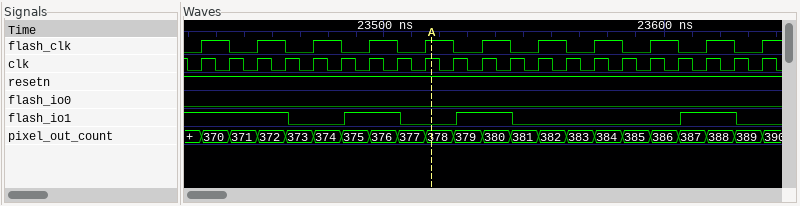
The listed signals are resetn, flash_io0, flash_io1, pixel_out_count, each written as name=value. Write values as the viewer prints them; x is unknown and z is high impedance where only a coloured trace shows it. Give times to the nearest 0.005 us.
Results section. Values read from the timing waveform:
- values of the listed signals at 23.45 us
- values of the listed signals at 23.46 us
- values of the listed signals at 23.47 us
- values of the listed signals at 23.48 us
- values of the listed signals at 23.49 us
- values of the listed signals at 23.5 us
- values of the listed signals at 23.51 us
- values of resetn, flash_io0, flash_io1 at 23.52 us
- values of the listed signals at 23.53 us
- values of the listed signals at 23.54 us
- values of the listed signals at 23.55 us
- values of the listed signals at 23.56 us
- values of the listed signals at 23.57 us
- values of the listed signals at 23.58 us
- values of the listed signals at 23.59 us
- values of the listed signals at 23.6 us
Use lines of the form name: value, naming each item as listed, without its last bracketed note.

values of the listed signals at 23.45 us: resetn=1, flash_io0=0, flash_io1=1, pixel_out_count=371
values of the listed signals at 23.46 us: resetn=1, flash_io0=0, flash_io1=1, pixel_out_count=372
values of the listed signals at 23.47 us: resetn=1, flash_io0=0, flash_io1=0, pixel_out_count=373
values of the listed signals at 23.48 us: resetn=1, flash_io0=0, flash_io1=0, pixel_out_count=374
values of the listed signals at 23.49 us: resetn=1, flash_io0=0, flash_io1=1, pixel_out_count=375
values of the listed signals at 23.5 us: resetn=1, flash_io0=0, flash_io1=1, pixel_out_count=376
values of the listed signals at 23.51 us: resetn=1, flash_io0=0, flash_io1=0, pixel_out_count=377
values of resetn, flash_io0, flash_io1 at 23.52 us: resetn=1, flash_io0=0, flash_io1=0
values of the listed signals at 23.53 us: resetn=1, flash_io0=0, flash_io1=1, pixel_out_count=379
values of the listed signals at 23.54 us: resetn=1, flash_io0=0, flash_io1=1, pixel_out_count=380
values of the listed signals at 23.55 us: resetn=1, flash_io0=0, flash_io1=0, pixel_out_count=381
values of the listed signals at 23.56 us: resetn=1, flash_io0=0, flash_io1=0, pixel_out_count=382
values of the listed signals at 23.57 us: resetn=1, flash_io0=0, flash_io1=0, pixel_out_count=383
values of the listed signals at 23.58 us: resetn=1, flash_io0=0, flash_io1=0, pixel_out_count=384
values of the listed signals at 23.59 us: resetn=1, flash_io0=0, flash_io1=0, pixel_out_count=385
values of the listed signals at 23.6 us: resetn=1, flash_io0=0, flash_io1=0, pixel_out_count=386
